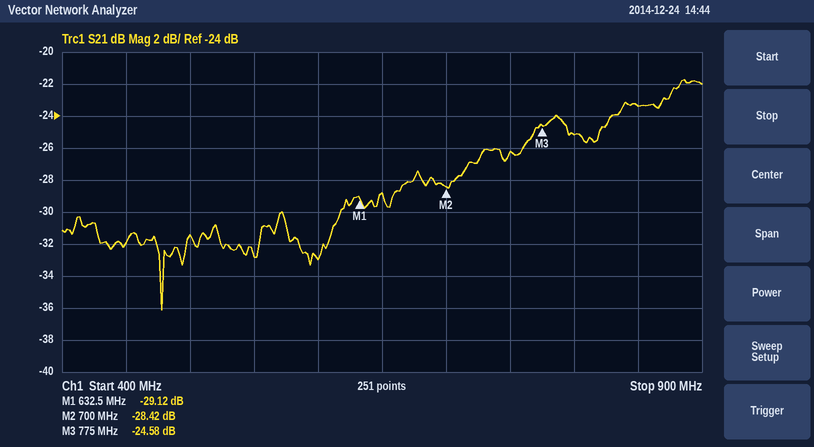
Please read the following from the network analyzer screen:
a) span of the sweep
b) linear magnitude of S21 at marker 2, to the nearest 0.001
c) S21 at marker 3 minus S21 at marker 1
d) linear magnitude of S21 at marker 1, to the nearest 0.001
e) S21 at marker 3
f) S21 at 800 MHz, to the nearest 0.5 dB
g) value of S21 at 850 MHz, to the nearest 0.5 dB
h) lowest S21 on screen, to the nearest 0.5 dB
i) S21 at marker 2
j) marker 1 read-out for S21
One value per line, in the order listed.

500 MHz
0.038
4.54 dB
0.035
-24.58 dB
-25.0 dB
-23.5 dB
-36.0 dB
-28.42 dB
-29.12 dB
